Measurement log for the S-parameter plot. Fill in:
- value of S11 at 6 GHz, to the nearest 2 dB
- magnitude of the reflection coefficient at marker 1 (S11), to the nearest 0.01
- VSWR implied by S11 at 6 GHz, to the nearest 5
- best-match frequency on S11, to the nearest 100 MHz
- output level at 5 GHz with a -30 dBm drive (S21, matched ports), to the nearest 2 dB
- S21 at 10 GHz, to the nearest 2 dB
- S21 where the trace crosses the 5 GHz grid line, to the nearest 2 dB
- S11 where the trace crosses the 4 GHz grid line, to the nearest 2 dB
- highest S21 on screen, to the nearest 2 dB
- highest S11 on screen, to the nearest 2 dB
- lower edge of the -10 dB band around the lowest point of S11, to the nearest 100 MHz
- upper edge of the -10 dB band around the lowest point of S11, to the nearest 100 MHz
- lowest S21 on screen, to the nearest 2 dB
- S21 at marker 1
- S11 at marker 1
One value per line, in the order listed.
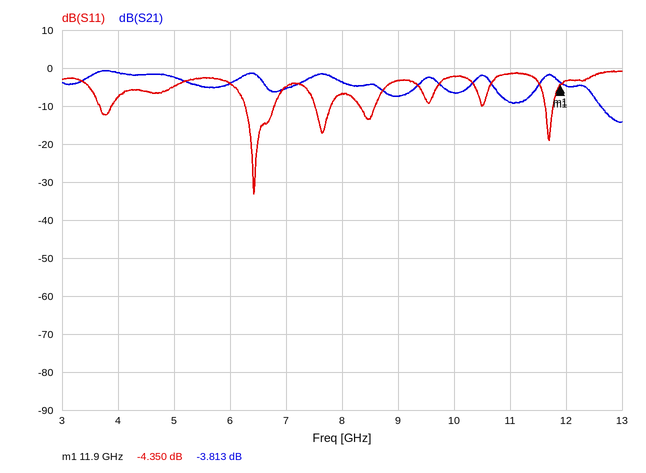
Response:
-4 dB
0.61
5
6.4 GHz
-32 dBm
-6 dB
-2 dB
-8 dB
0 dB
0 dB
6.3 GHz
6.8 GHz
-14 dB
-3.813 dB
-4.350 dB
